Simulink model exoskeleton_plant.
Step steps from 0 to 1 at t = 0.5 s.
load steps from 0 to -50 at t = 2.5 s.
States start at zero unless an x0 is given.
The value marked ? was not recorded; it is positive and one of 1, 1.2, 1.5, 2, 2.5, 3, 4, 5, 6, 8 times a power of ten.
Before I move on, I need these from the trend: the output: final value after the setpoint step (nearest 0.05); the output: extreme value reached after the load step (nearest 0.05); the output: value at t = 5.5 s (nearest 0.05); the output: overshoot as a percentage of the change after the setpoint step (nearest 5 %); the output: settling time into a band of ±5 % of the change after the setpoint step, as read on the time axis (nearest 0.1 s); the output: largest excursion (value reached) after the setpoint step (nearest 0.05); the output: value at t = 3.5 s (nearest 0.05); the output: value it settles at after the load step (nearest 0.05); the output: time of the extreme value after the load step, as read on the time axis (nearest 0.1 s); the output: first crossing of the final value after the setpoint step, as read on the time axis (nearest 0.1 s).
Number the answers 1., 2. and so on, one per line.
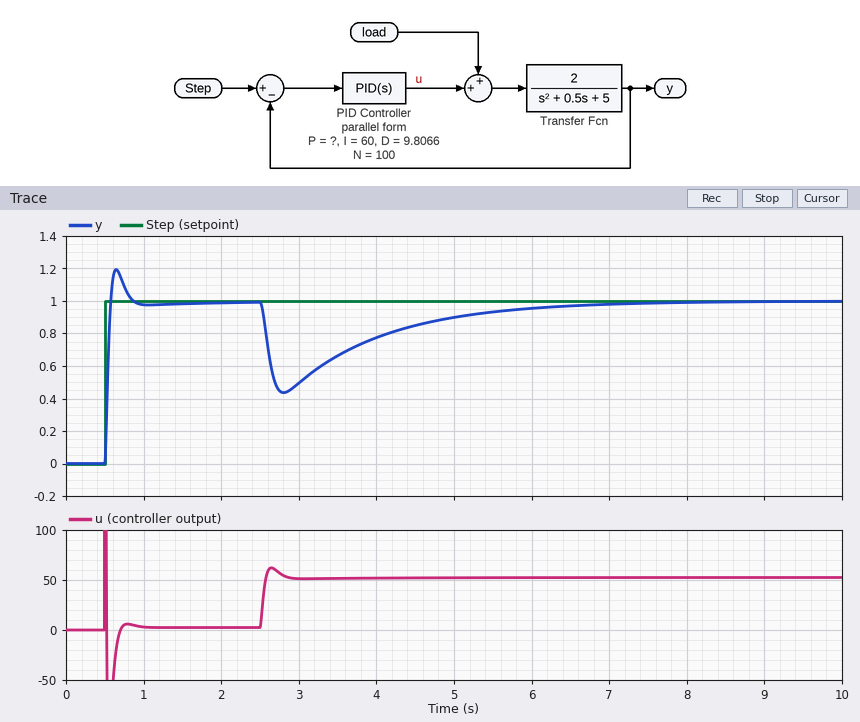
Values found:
1. 1.00
2. 0.45
3. 0.95
4. 20 %
5. 0.8 s
6. 1.20
7. 0.65
8. 1.00
9. 2.8 s
10. 0.6 s
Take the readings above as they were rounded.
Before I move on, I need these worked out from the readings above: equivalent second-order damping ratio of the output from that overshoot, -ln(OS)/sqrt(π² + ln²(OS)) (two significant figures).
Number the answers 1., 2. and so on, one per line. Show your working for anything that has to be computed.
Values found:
1. ln(0.2) = -1.609; 1.609 / sqrt(9.870 + 2.590) = 0.46
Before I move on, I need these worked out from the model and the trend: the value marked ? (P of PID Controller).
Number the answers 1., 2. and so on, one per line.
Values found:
1. 80
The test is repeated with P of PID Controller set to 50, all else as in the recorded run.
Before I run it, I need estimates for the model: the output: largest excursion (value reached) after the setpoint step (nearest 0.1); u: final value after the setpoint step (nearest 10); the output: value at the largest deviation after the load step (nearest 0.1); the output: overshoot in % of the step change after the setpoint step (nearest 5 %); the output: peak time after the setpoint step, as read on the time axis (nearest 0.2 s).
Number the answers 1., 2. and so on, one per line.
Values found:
1. 1.1
2. 0
3. 0.2
4. 15 %
5. 0.6 s
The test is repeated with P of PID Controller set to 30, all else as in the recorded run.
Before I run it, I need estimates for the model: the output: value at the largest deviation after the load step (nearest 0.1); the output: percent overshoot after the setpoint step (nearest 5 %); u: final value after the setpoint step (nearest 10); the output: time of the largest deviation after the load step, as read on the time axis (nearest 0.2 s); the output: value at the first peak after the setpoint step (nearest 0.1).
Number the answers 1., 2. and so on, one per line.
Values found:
1. 0.0
2. 10 %
3. 0
4. 3.0 s
5. 1.1
